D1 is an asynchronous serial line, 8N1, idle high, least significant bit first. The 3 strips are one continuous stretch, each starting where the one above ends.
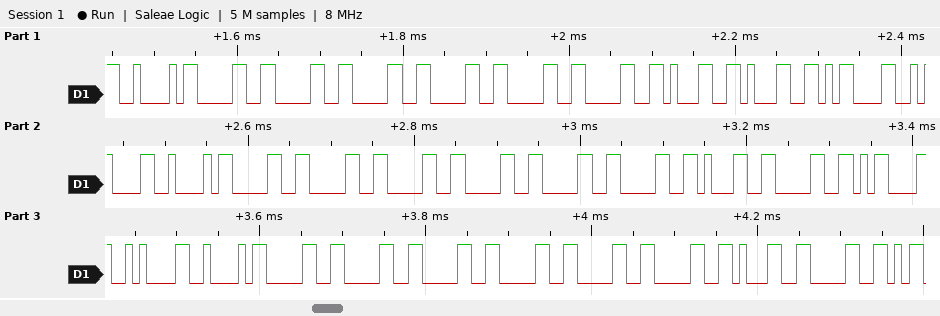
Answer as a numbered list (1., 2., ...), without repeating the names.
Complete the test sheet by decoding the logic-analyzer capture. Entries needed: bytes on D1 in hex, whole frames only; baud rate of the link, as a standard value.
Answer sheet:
1. 42 30 30 30 30 30 30 31 31 0D 0A 42 30 30 30 30 30 30 31 30 0D 0A 42 30 30 30 30 30 30 31 30
2. 115200 baud
